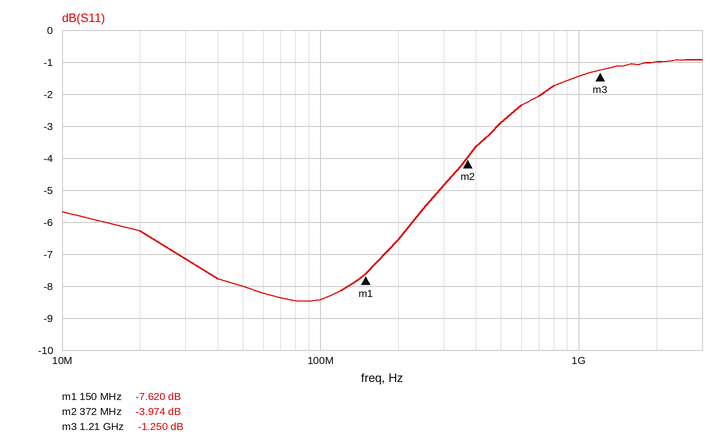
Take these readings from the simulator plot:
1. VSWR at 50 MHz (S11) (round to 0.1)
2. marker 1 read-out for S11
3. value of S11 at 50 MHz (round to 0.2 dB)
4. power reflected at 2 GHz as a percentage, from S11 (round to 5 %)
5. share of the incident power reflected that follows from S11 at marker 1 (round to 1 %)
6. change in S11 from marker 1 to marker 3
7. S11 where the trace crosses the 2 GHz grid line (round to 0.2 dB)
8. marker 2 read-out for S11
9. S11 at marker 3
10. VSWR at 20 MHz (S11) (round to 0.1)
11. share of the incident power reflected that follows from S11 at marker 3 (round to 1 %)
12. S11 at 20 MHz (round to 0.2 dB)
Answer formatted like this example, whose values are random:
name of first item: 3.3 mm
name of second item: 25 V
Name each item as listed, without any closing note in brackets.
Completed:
VSWR at 50 MHz (S11): 2.3
marker 1 read-out for S11: -7.620 dB
value of S11 at 50 MHz: -8.0 dB
power reflected at 2 GHz as a percentage, from S11: 80 %
share of the incident power reflected that follows from S11 at marker 1: 17 %
change in S11 from marker 1 to marker 3: 6.370 dB
S11 where the trace crosses the 2 GHz grid line: -1.0 dB
marker 2 read-out for S11: -3.974 dB
S11 at marker 3: -1.250 dB
VSWR at 20 MHz (S11): 2.9
share of the incident power reflected that follows from S11 at marker 3: 75 %
S11 at 20 MHz: -6.2 dB
